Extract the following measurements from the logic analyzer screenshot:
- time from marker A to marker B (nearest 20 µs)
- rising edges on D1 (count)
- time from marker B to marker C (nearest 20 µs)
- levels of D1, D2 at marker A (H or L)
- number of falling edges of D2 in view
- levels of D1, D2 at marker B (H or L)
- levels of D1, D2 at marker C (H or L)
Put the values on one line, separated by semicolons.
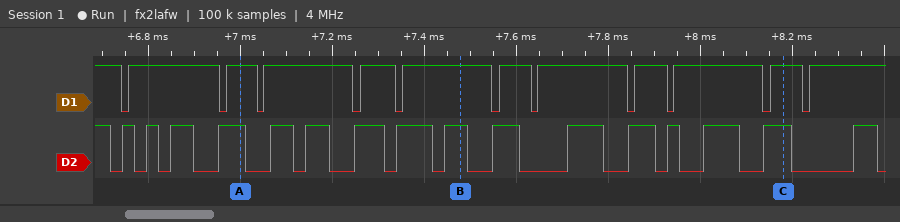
480 µs; 11; 700 µs; D1=H, D2=H; 17; D1=H, D2=H; D1=H, D2=H
